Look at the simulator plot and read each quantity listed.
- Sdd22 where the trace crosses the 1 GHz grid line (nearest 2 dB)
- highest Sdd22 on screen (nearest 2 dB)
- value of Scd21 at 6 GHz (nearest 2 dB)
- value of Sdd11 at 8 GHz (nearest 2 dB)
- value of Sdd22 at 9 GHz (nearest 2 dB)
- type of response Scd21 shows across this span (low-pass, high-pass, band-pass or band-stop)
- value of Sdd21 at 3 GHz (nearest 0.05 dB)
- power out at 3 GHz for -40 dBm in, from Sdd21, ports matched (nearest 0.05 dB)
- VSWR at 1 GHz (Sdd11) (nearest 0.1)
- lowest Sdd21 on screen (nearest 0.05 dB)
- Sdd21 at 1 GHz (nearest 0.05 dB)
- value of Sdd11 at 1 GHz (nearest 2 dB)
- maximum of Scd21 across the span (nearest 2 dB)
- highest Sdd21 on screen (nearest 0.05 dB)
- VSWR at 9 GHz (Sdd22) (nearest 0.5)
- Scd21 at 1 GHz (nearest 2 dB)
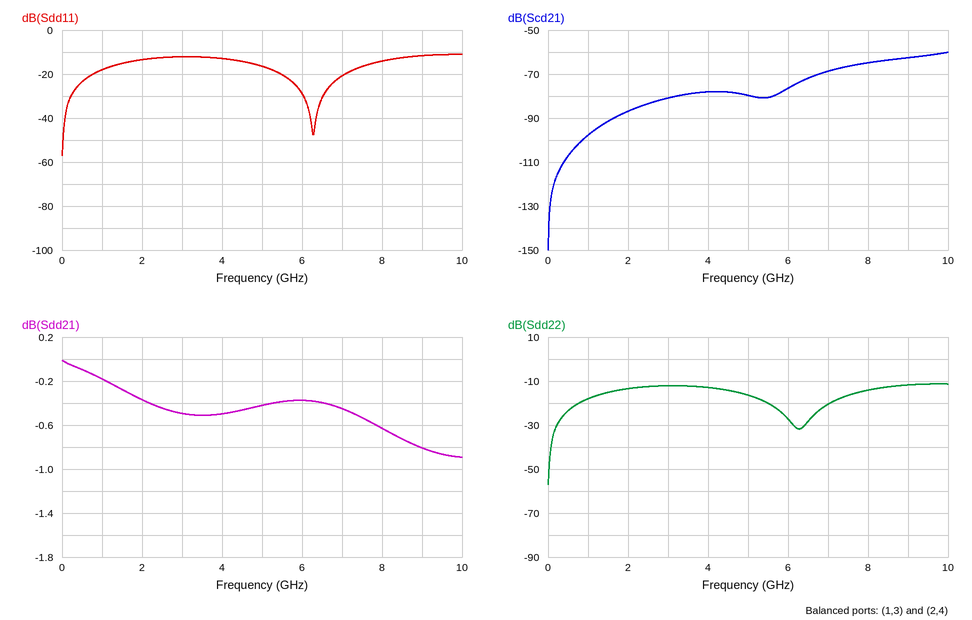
-18 dB
-12 dB
-76 dB
-14 dB
-12 dB
high-pass
-0.50 dB
-40.50 dBm
1.3
-0.90 dB
-0.20 dB
-18 dB
-60 dB
0.00 dB
1.5
-98 dB
